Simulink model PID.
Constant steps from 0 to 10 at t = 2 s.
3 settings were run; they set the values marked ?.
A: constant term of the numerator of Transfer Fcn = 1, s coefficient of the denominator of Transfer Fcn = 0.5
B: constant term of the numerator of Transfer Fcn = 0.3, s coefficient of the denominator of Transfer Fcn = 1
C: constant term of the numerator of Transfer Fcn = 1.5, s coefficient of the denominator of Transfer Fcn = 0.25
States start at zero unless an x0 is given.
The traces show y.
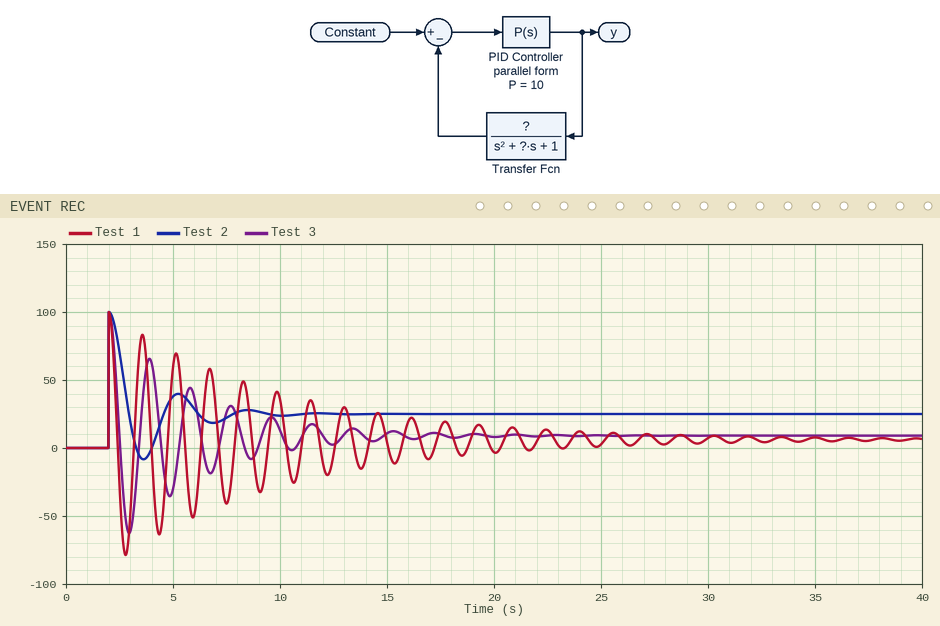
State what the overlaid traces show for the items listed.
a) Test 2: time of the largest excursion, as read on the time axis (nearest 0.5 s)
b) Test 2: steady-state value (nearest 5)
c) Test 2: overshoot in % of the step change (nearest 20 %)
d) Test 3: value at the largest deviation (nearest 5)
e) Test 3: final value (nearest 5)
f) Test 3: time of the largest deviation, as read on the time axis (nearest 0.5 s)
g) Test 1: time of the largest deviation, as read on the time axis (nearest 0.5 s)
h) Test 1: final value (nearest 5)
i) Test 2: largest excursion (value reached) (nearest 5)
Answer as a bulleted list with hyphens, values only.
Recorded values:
- 2.0 s
- 25
- 300 %
- 100
- 10
- 2.0 s
- 2.0 s
- 5
- 100
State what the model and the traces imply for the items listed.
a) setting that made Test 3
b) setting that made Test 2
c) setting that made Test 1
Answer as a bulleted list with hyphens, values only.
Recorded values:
- A
- B
- C
